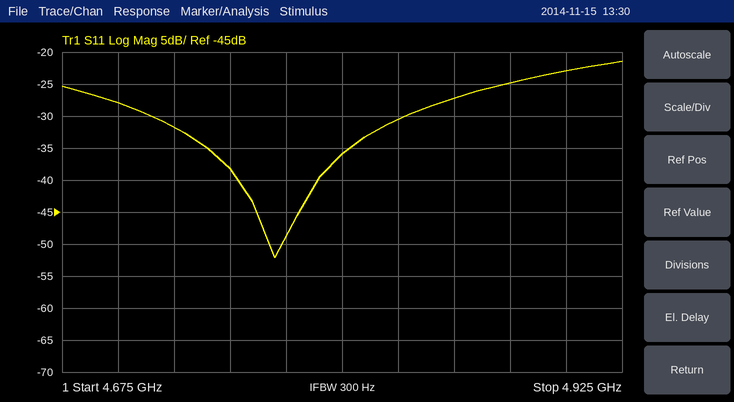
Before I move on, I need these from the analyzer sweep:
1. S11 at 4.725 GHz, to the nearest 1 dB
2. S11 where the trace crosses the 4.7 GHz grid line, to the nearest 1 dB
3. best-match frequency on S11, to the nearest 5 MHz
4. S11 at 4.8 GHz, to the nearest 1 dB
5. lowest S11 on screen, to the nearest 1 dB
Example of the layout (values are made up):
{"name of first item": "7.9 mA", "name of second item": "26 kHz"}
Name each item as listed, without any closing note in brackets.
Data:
{"S11 at 4.725 GHz, to the nearest 1 dB": "-32 dB", "S11 where the trace crosses the 4.7 GHz grid line, to the nearest 1 dB": "-28 dB", "best-match frequency on S11, to the nearest 5 MHz": "4.770 GHz", "S11 at 4.8 GHz, to the nearest 1 dB": "-36 dB", "lowest S11 on screen, to the nearest 1 dB": "-52 dB"}
